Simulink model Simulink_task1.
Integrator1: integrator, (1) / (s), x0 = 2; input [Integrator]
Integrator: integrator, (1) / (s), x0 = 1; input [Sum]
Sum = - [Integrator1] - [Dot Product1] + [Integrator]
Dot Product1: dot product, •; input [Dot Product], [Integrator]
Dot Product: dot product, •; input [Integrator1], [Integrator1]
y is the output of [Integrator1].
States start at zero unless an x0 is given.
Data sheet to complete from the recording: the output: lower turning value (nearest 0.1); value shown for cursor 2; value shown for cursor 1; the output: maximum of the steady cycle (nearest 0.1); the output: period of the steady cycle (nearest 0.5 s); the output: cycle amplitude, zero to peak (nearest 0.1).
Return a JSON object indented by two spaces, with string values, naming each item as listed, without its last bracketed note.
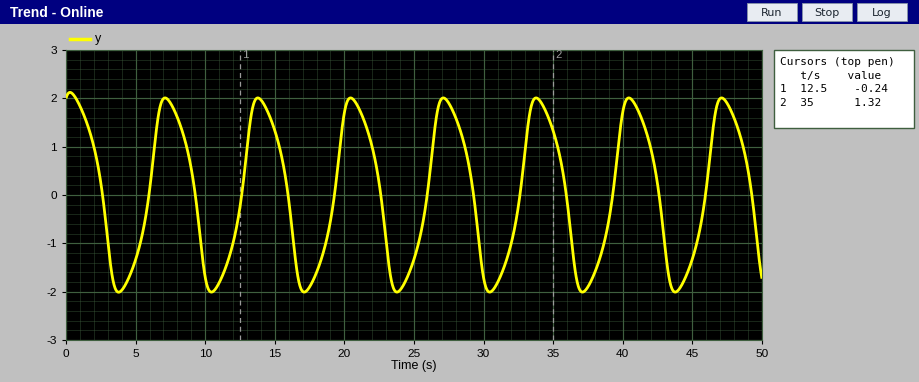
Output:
{
  "the output: lower turning value": "-2.0",
  "value shown for cursor 2": "1.32",
  "value shown for cursor 1": "-0.24",
  "the output: maximum of the steady cycle": "2.0",
  "the output: period of the steady cycle": "6.5 s",
  "the output: cycle amplitude, zero to peak": "2.0"
}
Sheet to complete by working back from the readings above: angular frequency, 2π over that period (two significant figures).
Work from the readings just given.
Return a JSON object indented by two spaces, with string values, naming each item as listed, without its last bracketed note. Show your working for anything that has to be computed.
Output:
{
  "angular frequency, 2π over that period": "2π / 6.5 = 0.97 rad/s"
}
